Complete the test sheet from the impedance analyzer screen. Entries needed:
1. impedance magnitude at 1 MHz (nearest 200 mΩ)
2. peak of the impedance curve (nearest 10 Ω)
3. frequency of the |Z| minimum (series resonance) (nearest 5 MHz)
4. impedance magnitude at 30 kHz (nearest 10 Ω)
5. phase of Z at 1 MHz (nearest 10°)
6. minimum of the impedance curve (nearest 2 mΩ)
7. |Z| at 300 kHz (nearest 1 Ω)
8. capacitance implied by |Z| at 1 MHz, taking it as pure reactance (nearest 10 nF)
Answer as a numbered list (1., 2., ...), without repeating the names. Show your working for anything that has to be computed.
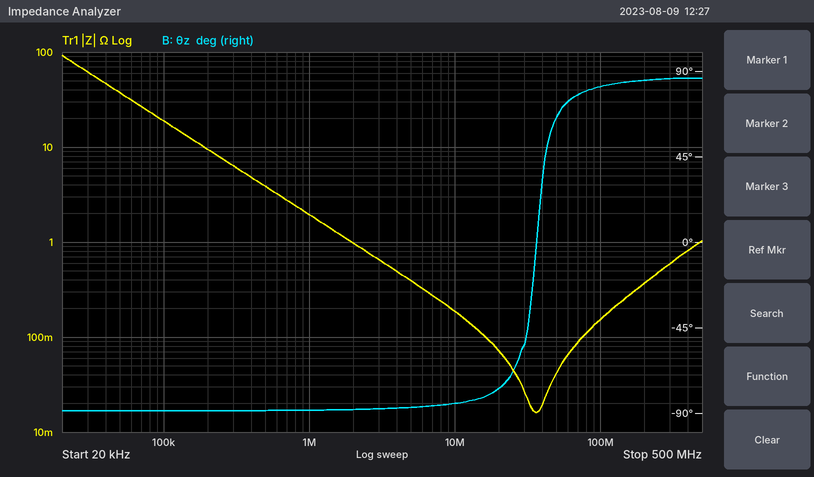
1. 2.0 Ω
2. 90 Ω
3. 35 MHz
4. 60 Ω
5. -90°
6. 16 mΩ
7. 6 Ω
8. C = 1/(2π × 1 MHz × 2.0 Ω) ≈ 80 nF
